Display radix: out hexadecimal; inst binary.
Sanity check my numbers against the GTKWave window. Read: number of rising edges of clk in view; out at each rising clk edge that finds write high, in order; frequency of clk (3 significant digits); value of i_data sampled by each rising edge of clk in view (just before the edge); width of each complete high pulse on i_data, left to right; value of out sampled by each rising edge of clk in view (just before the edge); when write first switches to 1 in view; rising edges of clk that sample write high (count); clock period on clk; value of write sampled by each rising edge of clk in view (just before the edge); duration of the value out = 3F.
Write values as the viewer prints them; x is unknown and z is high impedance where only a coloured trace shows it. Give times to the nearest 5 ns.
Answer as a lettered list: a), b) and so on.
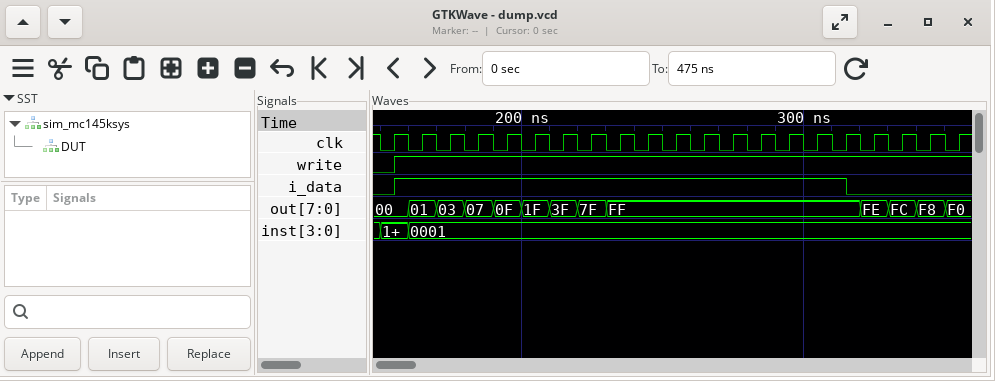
a) 21
b) 01, 03, 07, 0F, 1F, 3F, 7F, FF, FF, FF, FF, FF, FF, FF, FF, FF, FE, FC, F8, F0
c) 100 MHz
d) 0 1 1 1 1 1 1 1 1 1 1 1 1 1 1 1 1 0 0 0 0
e) 160 ns
f) 00, 01, 03, 07, 0F, 1F, 3F, 7F, FF, FF, FF, FF, FF, FF, FF, FF, FF, FE, FC, F8, F0
g) 155 ns
h) 20
i) 10 ns
j) 0 1 1 1 1 1 1 1 1 1 1 1 1 1 1 1 1 1 1 1 1
k) 10 ns
